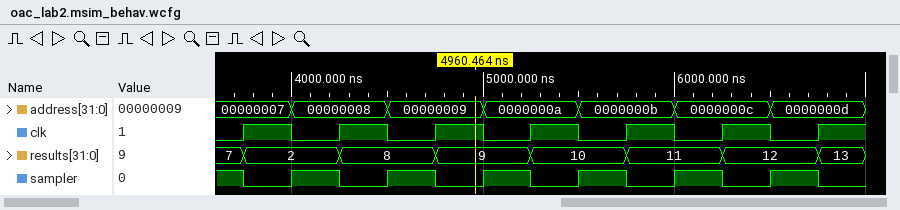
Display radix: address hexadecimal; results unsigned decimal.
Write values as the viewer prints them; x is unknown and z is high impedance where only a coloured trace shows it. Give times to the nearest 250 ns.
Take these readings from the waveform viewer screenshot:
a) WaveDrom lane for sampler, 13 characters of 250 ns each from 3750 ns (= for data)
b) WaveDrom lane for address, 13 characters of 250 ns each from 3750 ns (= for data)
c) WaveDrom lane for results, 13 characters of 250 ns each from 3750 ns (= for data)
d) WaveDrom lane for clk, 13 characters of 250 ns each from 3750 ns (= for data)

{name: 'sampler', wave: '0101010101010'}
{name: 'address', wave: '==.=.=.=.=.=.', data: '00000007 00000008 00000009 0000000a 0000000b 0000000c 0000000d'}
{name: 'results', wave: '=.=.=.=.=.=.=', data: '2 8 9 10 11 12 13'}
{name: 'clk', wave: '1010101010101'}
